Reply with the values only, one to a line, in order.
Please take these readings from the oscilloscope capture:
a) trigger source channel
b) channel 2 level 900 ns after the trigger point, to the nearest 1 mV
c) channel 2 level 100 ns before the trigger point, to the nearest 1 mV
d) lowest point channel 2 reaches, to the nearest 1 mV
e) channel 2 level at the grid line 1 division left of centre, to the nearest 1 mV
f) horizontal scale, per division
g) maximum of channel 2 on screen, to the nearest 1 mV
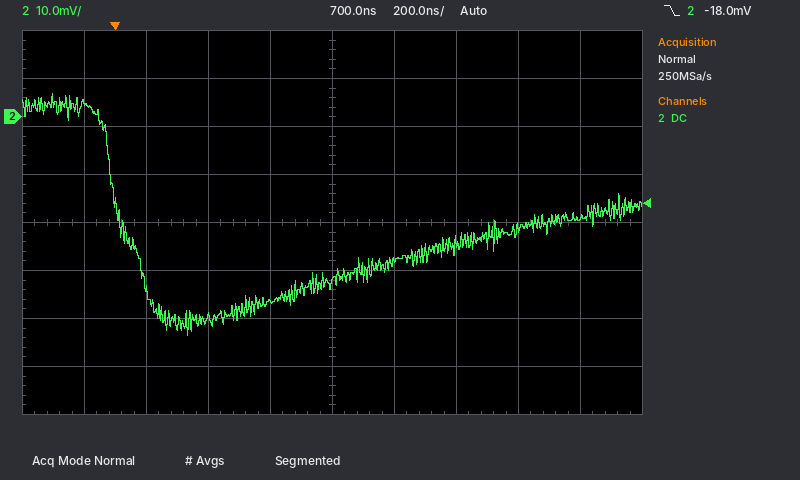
channel 2
-30 mV
3 mV
-46 mV
-38 mV
200 ns
5 mV
